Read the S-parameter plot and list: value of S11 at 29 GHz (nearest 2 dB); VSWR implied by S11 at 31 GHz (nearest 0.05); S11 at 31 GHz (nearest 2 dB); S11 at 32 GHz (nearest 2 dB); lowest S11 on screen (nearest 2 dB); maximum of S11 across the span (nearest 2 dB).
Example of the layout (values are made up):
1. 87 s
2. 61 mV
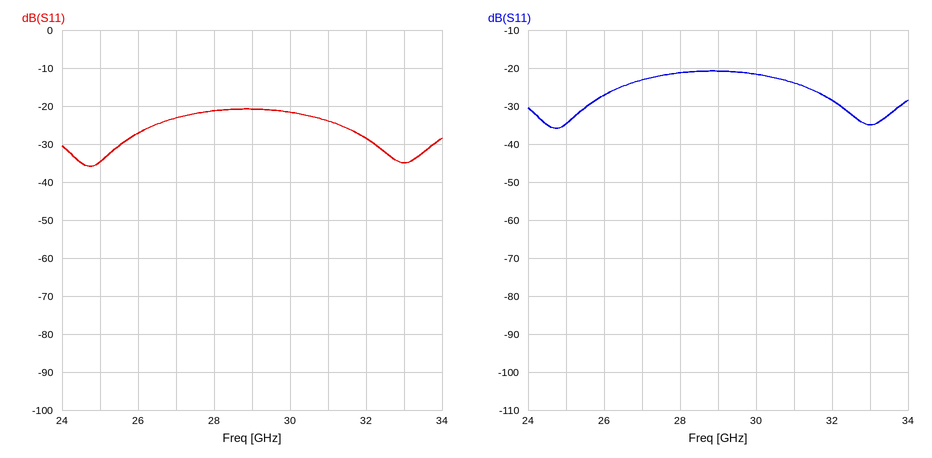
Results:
1. -20 dB
2. 1.15
3. -24 dB
4. -28 dB
5. -36 dB
6. -20 dB
